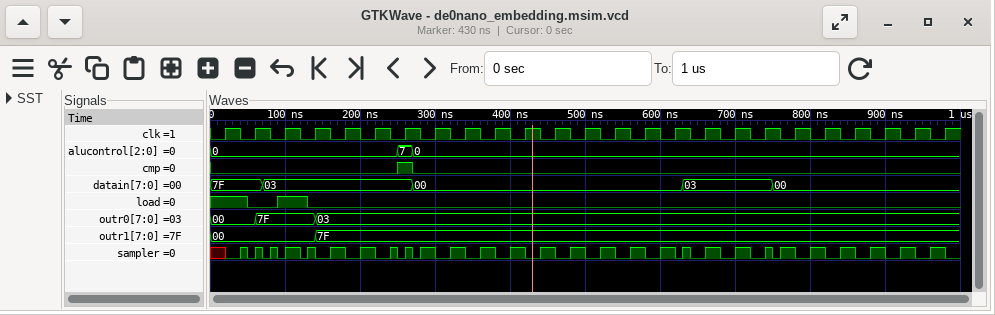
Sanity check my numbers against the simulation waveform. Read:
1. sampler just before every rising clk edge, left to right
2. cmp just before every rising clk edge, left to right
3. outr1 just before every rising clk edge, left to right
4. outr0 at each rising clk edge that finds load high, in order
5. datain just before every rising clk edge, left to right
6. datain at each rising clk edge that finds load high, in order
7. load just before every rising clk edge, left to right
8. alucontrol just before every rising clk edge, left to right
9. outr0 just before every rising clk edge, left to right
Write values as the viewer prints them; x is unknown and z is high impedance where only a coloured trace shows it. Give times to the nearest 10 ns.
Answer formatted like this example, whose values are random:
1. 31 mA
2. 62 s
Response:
1. x 0 0 1 1 1 0 1 1 1 1 1 1 1 1 1 0 0 0 1 1 1 1 1 1
2. 0 0 0 0 0 0 1 0 0 0 0 0 0 0 0 0 0 0 0 0 0 0 0 0 0
3. 00, 00, 00, 00, 7F, 7F, 7F, 7F, 7F, 7F, 7F, 7F, 7F, 7F, 7F, 7F, 7F, 7F, 7F, 7F, 7F, 7F, 7F, 7F, 7F
4. 00, 7F
5. 7F, 7F, 03, 03, 03, 03, 03, 00, 00, 00, 00, 00, 00, 00, 00, 00, 03, 03, 03, 00, 00, 00, 00, 00, 00
6. 7F, 03
7. 1 0 1 0 0 0 0 0 0 0 0 0 0 0 0 0 0 0 0 0 0 0 0 0 0
8. 0, 0, 0, 0, 0, 0, 7, 0, 0, 0, 0, 0, 0, 0, 0, 0, 0, 0, 0, 0, 0, 0, 0, 0, 0
9. 00, 00, 7F, 7F, 03, 03, 03, 03, 03, 03, 03, 03, 03, 03, 03, 03, 03, 03, 03, 03, 03, 03, 03, 03, 03
